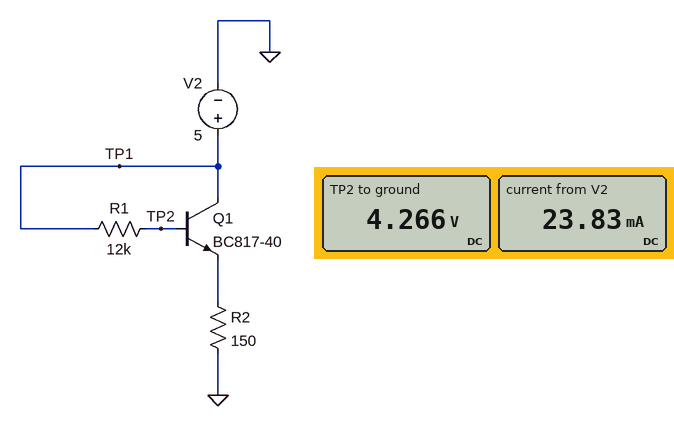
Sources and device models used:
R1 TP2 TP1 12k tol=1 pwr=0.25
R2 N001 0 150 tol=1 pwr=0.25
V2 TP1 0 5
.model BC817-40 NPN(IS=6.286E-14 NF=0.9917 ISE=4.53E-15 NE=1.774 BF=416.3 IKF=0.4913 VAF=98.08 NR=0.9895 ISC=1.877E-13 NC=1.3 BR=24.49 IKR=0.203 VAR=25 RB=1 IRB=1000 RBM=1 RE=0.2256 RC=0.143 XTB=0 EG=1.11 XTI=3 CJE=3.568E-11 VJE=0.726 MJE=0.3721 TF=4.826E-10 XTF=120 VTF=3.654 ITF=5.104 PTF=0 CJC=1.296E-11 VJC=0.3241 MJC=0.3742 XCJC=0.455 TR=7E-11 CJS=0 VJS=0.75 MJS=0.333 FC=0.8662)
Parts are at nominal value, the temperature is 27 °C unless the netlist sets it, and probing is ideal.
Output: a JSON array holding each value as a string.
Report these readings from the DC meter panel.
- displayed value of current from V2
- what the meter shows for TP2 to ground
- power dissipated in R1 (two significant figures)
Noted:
["23.83 mA", "4.266 V", "45 µW"]
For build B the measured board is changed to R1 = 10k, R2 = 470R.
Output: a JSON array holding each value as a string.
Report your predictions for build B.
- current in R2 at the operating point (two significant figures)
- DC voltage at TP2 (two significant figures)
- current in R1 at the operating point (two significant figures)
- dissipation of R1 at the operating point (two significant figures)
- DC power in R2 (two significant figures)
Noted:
["8.8 mA", "4.8 V", "22 µA", "4.8 µW", "36 mW"]
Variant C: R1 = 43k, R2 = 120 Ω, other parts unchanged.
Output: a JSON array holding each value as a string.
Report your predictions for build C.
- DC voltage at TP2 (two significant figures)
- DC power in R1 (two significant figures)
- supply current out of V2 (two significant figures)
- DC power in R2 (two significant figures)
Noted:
["3.0 V", "97 µW", "19 mA", "43 mW"]
